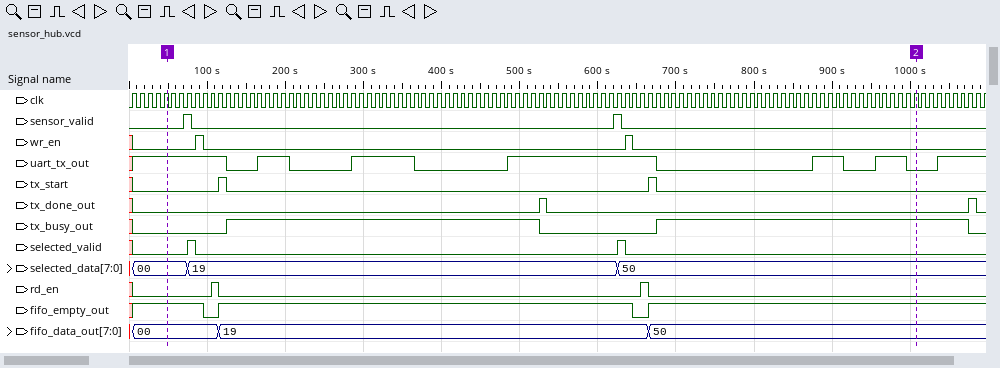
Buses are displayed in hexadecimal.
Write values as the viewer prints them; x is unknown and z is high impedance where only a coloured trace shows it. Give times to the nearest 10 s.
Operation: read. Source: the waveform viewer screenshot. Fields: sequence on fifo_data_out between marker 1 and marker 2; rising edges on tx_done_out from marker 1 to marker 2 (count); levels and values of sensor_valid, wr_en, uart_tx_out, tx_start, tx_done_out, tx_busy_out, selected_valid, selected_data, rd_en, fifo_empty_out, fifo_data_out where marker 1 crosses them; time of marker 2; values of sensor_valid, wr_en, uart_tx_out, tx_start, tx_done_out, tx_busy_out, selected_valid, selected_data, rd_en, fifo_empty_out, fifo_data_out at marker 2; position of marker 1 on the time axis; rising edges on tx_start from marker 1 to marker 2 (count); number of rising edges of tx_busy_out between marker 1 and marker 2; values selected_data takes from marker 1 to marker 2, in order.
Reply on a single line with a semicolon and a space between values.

00, 19, 50; 1; sensor_valid=0, wr_en=0, uart_tx_out=1, tx_start=0, tx_done_out=0, tx_busy_out=0, selected_valid=0, selected_data=00, rd_en=0, fifo_empty_out=1, fifo_data_out=00; 1010 s; sensor_valid=0, wr_en=0, uart_tx_out=0, tx_start=0, tx_done_out=0, tx_busy_out=1, selected_valid=0, selected_data=50, rd_en=0, fifo_empty_out=1, fifo_data_out=50; 50 s; 2; 2; 00, 19, 50
